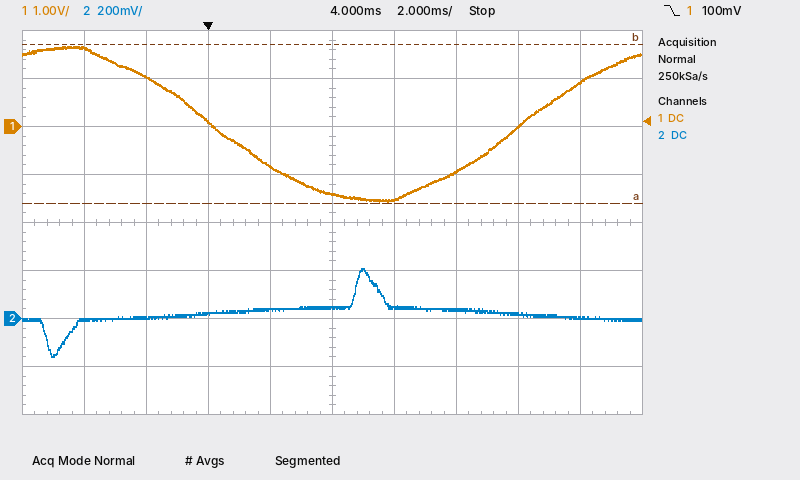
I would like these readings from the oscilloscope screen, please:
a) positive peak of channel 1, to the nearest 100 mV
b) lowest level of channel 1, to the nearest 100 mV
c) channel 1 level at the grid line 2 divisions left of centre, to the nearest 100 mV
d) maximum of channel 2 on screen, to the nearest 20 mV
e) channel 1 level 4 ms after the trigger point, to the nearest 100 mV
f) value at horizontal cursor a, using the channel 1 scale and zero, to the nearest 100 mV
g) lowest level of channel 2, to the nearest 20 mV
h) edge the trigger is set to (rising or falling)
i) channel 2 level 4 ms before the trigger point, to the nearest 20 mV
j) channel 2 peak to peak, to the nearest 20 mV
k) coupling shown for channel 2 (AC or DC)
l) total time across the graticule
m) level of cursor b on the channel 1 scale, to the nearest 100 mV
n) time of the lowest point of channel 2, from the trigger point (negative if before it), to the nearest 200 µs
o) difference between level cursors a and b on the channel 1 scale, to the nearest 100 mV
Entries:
1.7 V
-1.6 V
100 mV
200 mV
-1.4 V
-1.6 V
-160 mV
falling
0 mV
360 mV
DC
20 ms
1.7 V
-5.0 ms
3.3 V
